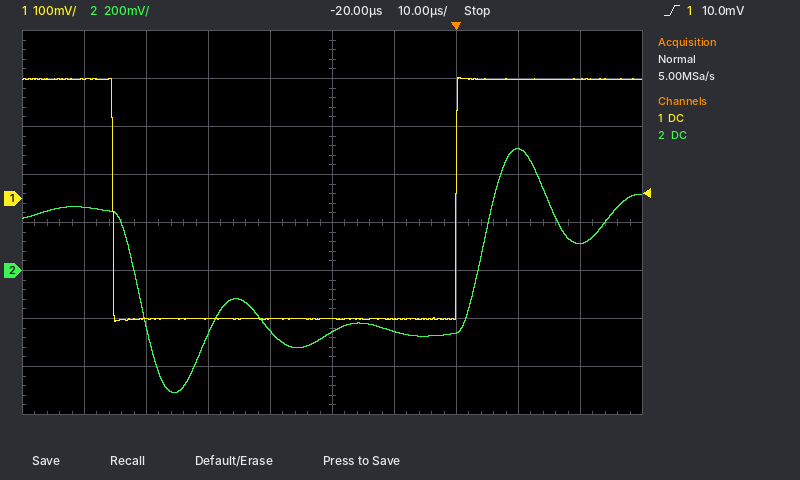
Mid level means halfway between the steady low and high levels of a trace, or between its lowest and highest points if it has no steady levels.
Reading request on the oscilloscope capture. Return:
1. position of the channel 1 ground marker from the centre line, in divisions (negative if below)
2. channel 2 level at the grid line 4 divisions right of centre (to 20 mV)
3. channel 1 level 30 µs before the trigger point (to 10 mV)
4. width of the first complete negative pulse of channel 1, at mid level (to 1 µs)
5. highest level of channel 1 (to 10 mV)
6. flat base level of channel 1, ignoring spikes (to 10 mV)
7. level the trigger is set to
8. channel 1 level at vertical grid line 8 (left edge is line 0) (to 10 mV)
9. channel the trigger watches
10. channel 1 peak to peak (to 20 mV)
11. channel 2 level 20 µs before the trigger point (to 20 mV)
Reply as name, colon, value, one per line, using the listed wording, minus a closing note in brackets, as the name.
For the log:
position of the channel 1 ground marker from the centre line, in divisions: +0.5 div
channel 2 level at the grid line 4 divisions right of centre: 120 mV
channel 1 level 30 µs before the trigger point: -250 mV
width of the first complete negative pulse of channel 1, at mid level: 55 µs
highest level of channel 1: 250 mV
flat base level of channel 1, ignoring spikes: -250 mV
level the trigger is set to: 10.0 mV
channel 1 level at vertical grid line 8 (left edge is line 0): 250 mV
channel the trigger watches: channel 1
channel 1 peak to peak: 500 mV
channel 2 level 20 µs before the trigger point: -260 mV
